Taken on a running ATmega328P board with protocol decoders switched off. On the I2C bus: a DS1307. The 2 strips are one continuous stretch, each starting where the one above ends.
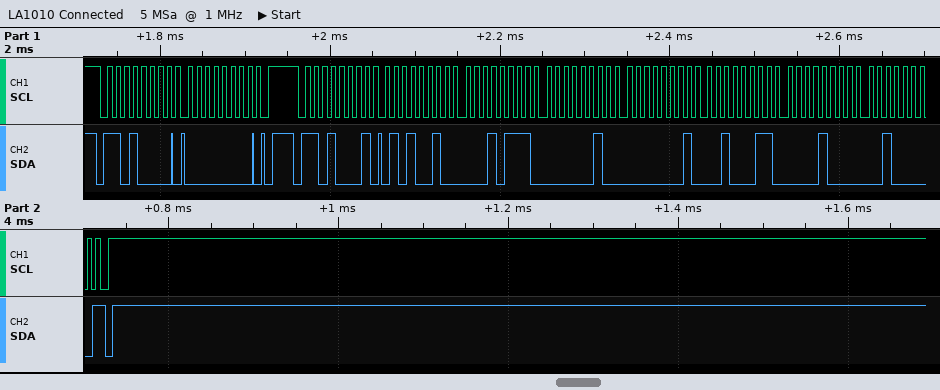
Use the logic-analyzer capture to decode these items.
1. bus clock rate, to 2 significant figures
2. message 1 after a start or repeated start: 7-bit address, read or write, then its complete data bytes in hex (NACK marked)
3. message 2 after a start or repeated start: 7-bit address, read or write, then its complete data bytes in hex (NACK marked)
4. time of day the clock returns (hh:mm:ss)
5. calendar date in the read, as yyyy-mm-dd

100 kHz
0x68 write: 00
0x68 read: 52 17 02 01 23 08 20 NACK
02:17:52
2020-08-23
